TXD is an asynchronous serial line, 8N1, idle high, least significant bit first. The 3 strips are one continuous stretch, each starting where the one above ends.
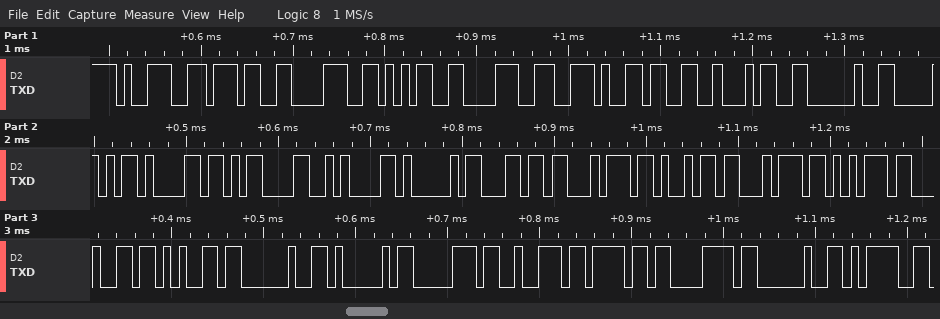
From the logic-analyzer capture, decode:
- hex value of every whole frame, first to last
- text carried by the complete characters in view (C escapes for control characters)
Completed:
0x39 0x37 0x38 0x35 0x38 0x2E 0x33 0x34 0x20 0x50 0x61 0x0D 0x0A 0x41 0x6C 0x74 0x69 0x74 0x75 0x64 0x65 0x20 0x41 0x70 0x72 0x6F 0x78 0x20 0x3D
"97858.34 Pa\r\nAltitude Aprox ="
